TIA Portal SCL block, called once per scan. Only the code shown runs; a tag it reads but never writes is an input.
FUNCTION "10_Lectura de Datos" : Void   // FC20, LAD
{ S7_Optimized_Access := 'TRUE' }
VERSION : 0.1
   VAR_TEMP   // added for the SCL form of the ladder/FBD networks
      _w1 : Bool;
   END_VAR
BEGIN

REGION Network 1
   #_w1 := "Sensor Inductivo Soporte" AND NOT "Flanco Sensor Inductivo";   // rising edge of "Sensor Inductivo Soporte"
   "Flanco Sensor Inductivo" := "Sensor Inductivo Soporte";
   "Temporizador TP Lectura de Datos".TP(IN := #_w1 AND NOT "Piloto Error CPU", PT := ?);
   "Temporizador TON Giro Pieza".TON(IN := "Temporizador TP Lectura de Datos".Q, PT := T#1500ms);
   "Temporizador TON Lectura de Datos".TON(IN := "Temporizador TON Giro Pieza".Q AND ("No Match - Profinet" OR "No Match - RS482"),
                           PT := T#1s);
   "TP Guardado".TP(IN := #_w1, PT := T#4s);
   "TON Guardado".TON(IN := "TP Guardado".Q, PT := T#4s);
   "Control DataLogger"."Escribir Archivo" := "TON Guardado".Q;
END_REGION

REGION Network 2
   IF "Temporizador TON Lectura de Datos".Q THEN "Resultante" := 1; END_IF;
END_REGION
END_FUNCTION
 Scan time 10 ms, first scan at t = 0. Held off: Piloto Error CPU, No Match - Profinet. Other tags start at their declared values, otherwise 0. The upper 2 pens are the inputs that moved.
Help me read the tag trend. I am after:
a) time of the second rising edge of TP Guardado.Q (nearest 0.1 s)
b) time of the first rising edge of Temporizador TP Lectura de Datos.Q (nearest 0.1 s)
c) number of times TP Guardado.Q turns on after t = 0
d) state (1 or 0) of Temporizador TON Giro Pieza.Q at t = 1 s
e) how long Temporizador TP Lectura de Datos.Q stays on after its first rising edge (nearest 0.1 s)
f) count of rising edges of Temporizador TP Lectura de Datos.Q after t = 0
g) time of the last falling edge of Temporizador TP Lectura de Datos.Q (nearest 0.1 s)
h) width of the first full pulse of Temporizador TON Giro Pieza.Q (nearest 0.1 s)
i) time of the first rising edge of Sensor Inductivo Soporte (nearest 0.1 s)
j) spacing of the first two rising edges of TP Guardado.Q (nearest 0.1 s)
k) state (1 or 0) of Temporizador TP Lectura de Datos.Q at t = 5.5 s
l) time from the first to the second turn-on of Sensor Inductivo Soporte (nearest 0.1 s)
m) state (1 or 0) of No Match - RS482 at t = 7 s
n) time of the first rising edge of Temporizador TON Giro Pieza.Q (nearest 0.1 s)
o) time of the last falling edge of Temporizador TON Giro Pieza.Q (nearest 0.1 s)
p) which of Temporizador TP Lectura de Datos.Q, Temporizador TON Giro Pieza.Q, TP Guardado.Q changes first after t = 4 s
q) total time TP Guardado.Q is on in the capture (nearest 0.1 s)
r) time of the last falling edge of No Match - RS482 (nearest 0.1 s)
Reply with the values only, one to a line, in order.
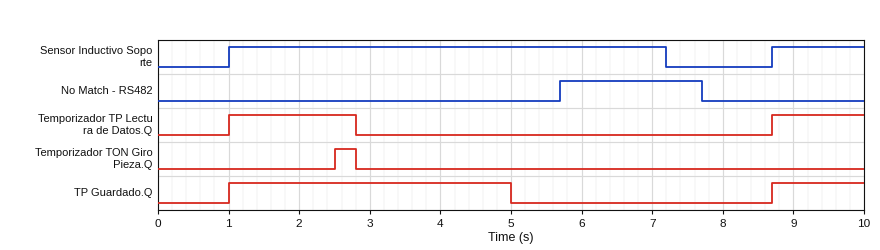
8.7 s
1.0 s
2
0
1.8 s
2
2.8 s
0.3 s
1.0 s
7.7 s
0
7.7 s
1
2.5 s
2.8 s
TP Guardado.Q
5.3 s
7.7 s
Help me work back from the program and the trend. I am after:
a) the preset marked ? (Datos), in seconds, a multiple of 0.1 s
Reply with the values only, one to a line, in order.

1.8 s
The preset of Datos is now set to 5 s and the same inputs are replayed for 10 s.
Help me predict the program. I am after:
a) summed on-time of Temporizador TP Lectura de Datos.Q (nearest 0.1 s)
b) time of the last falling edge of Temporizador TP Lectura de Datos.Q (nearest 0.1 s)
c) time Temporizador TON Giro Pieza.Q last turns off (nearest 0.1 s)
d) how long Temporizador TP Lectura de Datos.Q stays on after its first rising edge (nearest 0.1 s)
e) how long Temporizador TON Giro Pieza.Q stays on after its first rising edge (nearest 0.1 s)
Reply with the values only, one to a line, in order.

6.3 s
6.0 s
6.0 s
5.0 s
3.5 s
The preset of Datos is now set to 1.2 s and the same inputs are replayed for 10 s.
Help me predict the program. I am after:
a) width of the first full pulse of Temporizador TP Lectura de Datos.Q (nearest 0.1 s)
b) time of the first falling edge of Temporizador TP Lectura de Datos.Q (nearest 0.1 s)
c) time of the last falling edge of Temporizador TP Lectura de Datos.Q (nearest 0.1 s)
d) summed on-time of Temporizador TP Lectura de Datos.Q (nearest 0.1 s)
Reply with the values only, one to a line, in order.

1.2 s
2.2 s
9.9 s
2.4 s
